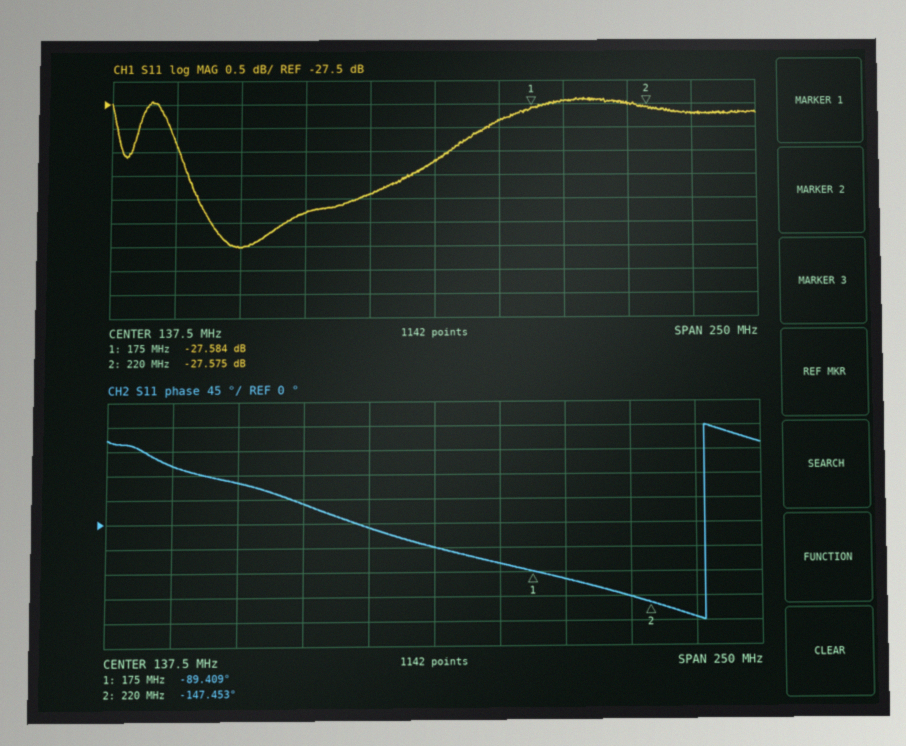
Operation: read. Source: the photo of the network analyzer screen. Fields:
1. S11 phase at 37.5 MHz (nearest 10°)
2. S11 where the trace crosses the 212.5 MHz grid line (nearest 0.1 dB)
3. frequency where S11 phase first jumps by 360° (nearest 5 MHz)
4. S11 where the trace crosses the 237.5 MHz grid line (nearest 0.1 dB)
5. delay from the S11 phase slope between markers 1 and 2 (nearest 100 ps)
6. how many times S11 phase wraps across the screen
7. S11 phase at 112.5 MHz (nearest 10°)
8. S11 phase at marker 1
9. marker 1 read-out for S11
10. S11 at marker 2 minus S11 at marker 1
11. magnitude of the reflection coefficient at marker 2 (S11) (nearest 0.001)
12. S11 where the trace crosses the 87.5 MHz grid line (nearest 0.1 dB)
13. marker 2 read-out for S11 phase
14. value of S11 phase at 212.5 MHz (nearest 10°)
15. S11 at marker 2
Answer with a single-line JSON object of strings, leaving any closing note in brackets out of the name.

{"S11 phase at 37.5 MHz": "110°", "S11 where the trace crosses the 212.5 MHz grid line": "-27.5 dB", "frequency where S11 phase first jumps by 360°": "240 MHz", "S11 where the trace crosses the 237.5 MHz grid line": "-27.7 dB", "delay from the S11 phase slope between markers 1 and 2": "3.6 ns", "how many times S11 phase wraps across the screen": "1", "S11 phase at 112.5 MHz": "-10°", "S11 phase at marker 1": "-89.409°", "marker 1 read-out for S11": "-27.584 dB", "S11 at marker 2 minus S11 at marker 1": "0.009 dB", "magnitude of the reflection coefficient at marker 2 (S11)": "0.042", "S11 where the trace crosses the 87.5 MHz grid line": "-29.8 dB", "marker 2 read-out for S11 phase": "-147.453°", "value of S11 phase at 212.5 MHz": "-140°", "S11 at marker 2": "-27.575 dB"}
